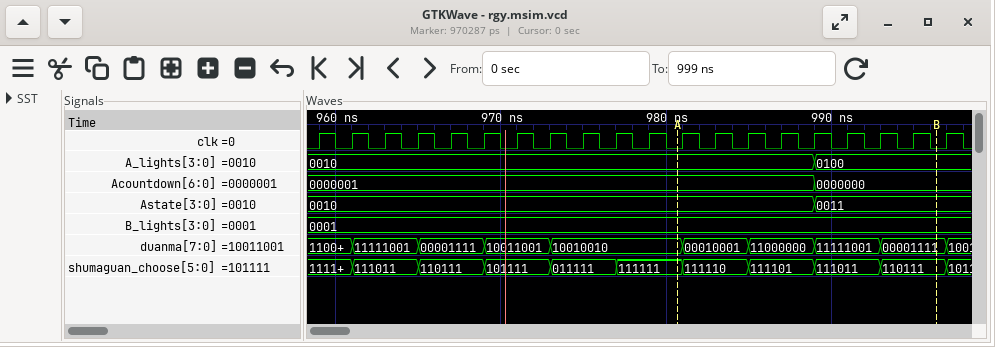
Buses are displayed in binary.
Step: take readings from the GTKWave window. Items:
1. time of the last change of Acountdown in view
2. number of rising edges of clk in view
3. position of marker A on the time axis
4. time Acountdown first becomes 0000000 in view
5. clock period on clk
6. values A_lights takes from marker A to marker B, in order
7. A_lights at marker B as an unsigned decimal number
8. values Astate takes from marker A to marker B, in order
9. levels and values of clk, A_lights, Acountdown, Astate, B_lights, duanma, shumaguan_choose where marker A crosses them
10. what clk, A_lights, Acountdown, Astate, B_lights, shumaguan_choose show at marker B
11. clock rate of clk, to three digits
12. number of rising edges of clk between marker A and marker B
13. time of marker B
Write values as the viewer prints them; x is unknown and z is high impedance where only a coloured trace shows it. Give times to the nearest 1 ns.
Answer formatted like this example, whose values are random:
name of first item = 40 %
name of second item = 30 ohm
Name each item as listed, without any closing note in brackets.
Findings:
time of the last change of Acountdown in view = 989 ns
number of rising edges of clk in view = 20
position of marker A on the time axis = 981 ns
time Acountdown first becomes 0000000 in view = 989 ns
clock period on clk = 2 ns
values A_lights takes from marker A to marker B, in order = 0010, 0100
A_lights at marker B as an unsigned decimal number = 4
values Astate takes from marker A to marker B, in order = 0010, 0011
levels and values of clk, A_lights, Acountdown, Astate, B_lights, duanma, shumaguan_choose where marker A crosses them = clk=0, A_lights=0010, Acountdown=0000001, Astate=0010, B_lights=0001, duanma=10010010, shumaguan_choose=111111
what clk, A_lights, Acountdown, Astate, B_lights, shumaguan_choose show at marker B = clk=0, A_lights=0100, Acountdown=0000000, Astate=0011, B_lights=0001, shumaguan_choose=110111
clock rate of clk, to three digits = 500 MHz
number of rising edges of clk between marker A and marker B = 8
time of marker B = 996 ns
